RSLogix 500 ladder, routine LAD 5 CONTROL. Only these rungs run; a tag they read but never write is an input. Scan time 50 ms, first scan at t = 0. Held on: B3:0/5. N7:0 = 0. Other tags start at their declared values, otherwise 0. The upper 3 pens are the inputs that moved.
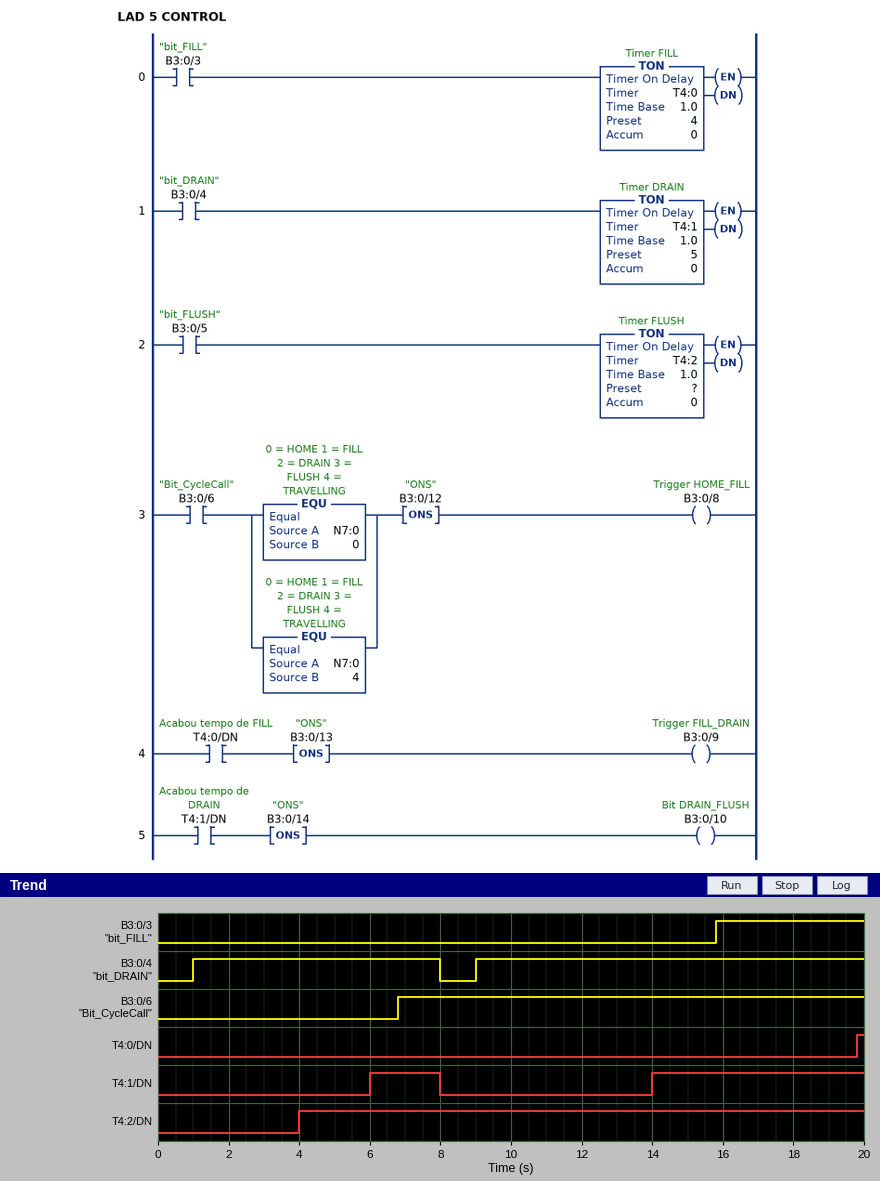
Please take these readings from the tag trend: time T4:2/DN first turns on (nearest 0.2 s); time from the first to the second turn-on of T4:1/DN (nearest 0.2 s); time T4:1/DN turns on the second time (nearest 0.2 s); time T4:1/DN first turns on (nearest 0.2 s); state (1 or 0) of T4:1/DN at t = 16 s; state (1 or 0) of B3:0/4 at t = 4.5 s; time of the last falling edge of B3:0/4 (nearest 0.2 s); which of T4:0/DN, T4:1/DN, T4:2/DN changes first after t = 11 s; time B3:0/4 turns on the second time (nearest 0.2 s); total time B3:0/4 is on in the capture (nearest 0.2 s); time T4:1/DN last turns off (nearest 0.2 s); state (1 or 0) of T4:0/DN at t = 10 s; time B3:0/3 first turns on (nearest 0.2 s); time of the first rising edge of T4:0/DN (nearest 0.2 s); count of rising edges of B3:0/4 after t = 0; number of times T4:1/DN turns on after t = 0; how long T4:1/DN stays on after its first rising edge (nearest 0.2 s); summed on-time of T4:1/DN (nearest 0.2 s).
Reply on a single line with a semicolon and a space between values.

4.0 s; 8.0 s; 14.0 s; 6.0 s; 1; 1; 8.0 s; T4:1/DN; 9.0 s; 18.0 s; 8.0 s; 0; 15.8 s; 19.8 s; 2; 2; 2.0 s; 8.0 s
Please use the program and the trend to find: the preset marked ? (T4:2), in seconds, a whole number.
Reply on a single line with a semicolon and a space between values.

4 s
